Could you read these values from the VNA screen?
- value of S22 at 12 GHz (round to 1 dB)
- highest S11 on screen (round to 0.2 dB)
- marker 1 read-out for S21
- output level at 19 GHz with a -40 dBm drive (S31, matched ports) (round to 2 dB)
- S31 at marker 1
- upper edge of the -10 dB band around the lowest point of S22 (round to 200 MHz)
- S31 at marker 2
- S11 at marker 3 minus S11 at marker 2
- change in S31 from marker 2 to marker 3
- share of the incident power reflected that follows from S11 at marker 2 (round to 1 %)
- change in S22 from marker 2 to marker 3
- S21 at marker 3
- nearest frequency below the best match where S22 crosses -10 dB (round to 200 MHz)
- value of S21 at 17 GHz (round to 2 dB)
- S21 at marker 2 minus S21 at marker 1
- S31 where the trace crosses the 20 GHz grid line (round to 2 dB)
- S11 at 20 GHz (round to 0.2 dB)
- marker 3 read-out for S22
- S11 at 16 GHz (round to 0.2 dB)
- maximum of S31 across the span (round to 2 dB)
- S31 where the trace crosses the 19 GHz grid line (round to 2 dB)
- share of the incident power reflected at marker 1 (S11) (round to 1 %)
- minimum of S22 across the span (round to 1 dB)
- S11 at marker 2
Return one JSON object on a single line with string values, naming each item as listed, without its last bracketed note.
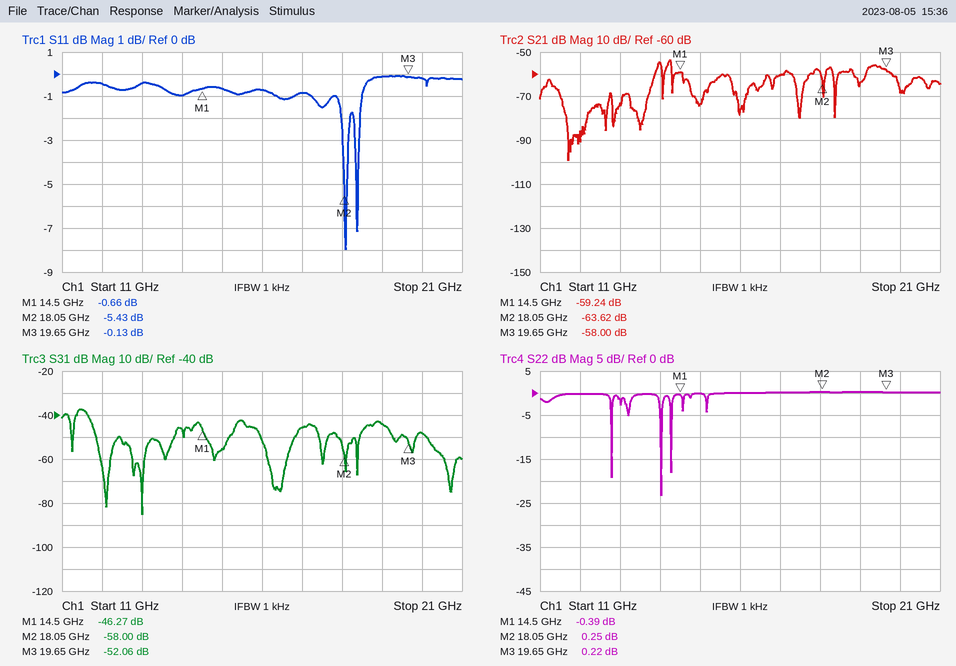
{"value of S22 at 12 GHz": "0 dB", "highest S11 on screen": "0.0 dB", "marker 1 read-out for S21": "-59.24 dB", "output level at 19 GHz with a -40 dBm drive (S31, matched ports)": "-84 dBm", "S31 at marker 1": "-46.27 dB", "upper edge of the -10 dB band around the lowest point of S22": "14.0 GHz", "S31 at marker 2": "-58.00 dB", "S11 at marker 3 minus S11 at marker 2": "5.30 dB", "change in S31 from marker 2 to marker 3": "5.94 dB", "share of the incident power reflected that follows from S11 at marker 2": "29 %", "change in S22 from marker 2 to marker 3": "-0.03 dB", "S21 at marker 3": "-58.00 dB", "nearest frequency below the best match where S22 crosses -10 dB": "14.0 GHz", "value of S21 at 17 GHz": "-60 dB", "S21 at marker 2 minus S21 at marker 1": "-4.38 dB", "S31 where the trace crosses the 20 GHz grid line": "-48 dB", "S11 at 20 GHz": "-0.2 dB", "marker 3 read-out for S22": "0.22 dB", "S11 at 16 GHz": "-0.8 dB", "maximum of S31 across the span": "-38 dB", "S31 where the trace crosses the 19 GHz grid line": "-44 dB", "share of the incident power reflected at marker 1 (S11)": "86 %", "minimum of S22 across the span": "-23 dB", "S11 at marker 2": "-5.43 dB"}
